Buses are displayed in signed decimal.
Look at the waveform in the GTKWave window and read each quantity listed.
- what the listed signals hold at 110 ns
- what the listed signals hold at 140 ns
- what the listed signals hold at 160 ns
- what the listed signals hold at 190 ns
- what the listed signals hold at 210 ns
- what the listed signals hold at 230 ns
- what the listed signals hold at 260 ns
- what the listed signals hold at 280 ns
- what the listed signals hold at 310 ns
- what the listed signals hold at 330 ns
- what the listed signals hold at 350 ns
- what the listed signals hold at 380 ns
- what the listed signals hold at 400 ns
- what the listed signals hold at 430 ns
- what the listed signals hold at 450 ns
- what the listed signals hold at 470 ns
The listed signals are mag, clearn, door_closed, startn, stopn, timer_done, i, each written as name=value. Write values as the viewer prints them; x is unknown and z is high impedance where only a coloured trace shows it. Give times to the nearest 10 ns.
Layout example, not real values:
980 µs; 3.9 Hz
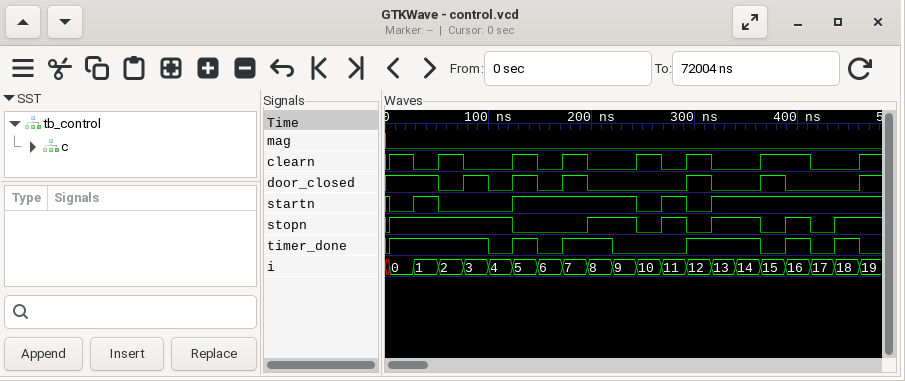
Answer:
mag=0, clearn=0, door_closed=0, startn=0, stopn=1, timer_done=0, i=4; mag=0, clearn=1, door_closed=1, startn=1, stopn=0, timer_done=1, i=5; mag=0, clearn=0, door_closed=0, startn=1, stopn=0, timer_done=0, i=6; mag=0, clearn=1, door_closed=1, startn=1, stopn=0, timer_done=1, i=7; mag=0, clearn=0, door_closed=0, startn=1, stopn=1, timer_done=1, i=8; mag=0, clearn=0, door_closed=0, startn=1, stopn=1, timer_done=0, i=9; mag=0, clearn=1, door_closed=0, startn=0, stopn=0, timer_done=0, i=10; mag=0, clearn=0, door_closed=0, startn=1, stopn=1, timer_done=0, i=11; mag=0, clearn=1, door_closed=1, startn=0, stopn=0, timer_done=1, i=12; mag=0, clearn=0, door_closed=0, startn=1, stopn=1, timer_done=1, i=13; mag=0, clearn=0, door_closed=0, startn=1, stopn=1, timer_done=1, i=14; mag=0, clearn=1, door_closed=1, startn=1, stopn=0, timer_done=0, i=15; mag=0, clearn=1, door_closed=0, startn=1, stopn=1, timer_done=1, i=16; mag=0, clearn=0, door_closed=0, startn=1, stopn=0, timer_done=0, i=17; mag=0, clearn=0, door_closed=0, startn=1, stopn=1, timer_done=1, i=18; mag=0, clearn=1, door_closed=1, startn=1, stopn=1, timer_done=0, i=19
